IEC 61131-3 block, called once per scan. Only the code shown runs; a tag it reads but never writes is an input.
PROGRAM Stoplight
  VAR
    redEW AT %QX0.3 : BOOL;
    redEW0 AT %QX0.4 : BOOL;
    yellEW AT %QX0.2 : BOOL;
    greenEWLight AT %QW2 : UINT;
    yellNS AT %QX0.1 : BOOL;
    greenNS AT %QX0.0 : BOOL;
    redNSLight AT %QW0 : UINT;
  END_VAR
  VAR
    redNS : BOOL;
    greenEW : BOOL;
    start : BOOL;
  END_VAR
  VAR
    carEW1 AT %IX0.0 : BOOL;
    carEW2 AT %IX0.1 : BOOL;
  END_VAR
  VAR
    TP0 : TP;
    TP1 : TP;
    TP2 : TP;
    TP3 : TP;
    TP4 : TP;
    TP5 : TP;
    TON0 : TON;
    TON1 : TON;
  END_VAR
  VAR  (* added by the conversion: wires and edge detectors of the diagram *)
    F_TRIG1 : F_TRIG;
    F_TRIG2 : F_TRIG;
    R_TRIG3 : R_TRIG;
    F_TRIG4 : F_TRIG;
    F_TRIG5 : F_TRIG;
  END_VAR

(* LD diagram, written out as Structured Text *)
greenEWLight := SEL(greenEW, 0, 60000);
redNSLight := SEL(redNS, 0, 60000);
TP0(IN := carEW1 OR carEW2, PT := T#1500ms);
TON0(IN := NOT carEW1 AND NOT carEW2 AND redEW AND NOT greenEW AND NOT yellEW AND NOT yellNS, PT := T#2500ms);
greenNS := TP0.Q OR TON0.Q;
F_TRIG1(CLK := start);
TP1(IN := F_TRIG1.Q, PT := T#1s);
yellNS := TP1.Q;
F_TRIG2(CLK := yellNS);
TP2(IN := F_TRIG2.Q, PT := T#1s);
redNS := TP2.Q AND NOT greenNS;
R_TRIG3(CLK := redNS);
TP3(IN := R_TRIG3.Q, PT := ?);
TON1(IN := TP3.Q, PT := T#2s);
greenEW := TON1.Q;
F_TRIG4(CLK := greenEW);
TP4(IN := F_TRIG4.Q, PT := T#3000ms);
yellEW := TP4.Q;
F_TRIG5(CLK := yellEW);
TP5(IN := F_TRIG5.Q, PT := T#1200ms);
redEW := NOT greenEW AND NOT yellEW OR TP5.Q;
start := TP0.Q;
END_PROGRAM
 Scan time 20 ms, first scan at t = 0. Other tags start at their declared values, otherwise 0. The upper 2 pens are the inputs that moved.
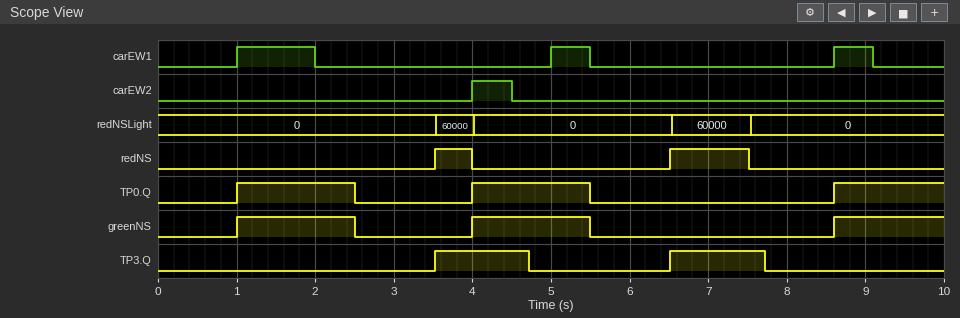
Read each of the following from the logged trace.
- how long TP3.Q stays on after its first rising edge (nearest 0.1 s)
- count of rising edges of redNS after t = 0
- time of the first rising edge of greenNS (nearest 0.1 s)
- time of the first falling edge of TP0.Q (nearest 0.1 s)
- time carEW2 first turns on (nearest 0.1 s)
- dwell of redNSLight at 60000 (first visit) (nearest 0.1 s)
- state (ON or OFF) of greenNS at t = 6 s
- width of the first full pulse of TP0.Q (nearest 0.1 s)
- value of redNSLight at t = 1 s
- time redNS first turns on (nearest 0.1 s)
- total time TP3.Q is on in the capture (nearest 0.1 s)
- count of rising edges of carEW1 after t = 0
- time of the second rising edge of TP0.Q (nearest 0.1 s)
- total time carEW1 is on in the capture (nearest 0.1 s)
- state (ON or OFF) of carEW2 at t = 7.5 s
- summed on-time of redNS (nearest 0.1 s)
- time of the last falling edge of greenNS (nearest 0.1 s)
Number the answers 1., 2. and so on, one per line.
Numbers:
1. 1.2 s
2. 2
3. 1.0 s
4. 2.5 s
5. 4.0 s
6. 0.5 s
7. OFF
8. 1.5 s
9. 0
10. 3.5 s
11. 2.4 s
12. 3
13. 4.0 s
14. 2.0 s
15. OFF
16. 1.5 s
17. 5.5 s
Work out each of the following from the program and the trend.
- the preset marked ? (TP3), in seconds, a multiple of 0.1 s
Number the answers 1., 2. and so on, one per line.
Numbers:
1. 1.2 s
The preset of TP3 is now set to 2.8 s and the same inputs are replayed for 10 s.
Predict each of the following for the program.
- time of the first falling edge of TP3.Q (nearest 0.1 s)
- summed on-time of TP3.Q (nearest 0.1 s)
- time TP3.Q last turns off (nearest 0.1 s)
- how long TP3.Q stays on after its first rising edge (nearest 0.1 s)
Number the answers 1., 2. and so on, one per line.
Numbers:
1. 6.3 s
2. 5.6 s
3. 9.3 s
4. 2.8 s
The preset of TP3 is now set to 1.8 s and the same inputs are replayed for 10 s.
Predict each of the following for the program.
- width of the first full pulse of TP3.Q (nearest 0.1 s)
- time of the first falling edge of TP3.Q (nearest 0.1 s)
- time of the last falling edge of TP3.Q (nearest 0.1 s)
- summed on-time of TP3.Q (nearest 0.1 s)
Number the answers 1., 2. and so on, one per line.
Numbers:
1. 1.8 s
2. 5.3 s
3. 8.3 s
4. 3.6 s
